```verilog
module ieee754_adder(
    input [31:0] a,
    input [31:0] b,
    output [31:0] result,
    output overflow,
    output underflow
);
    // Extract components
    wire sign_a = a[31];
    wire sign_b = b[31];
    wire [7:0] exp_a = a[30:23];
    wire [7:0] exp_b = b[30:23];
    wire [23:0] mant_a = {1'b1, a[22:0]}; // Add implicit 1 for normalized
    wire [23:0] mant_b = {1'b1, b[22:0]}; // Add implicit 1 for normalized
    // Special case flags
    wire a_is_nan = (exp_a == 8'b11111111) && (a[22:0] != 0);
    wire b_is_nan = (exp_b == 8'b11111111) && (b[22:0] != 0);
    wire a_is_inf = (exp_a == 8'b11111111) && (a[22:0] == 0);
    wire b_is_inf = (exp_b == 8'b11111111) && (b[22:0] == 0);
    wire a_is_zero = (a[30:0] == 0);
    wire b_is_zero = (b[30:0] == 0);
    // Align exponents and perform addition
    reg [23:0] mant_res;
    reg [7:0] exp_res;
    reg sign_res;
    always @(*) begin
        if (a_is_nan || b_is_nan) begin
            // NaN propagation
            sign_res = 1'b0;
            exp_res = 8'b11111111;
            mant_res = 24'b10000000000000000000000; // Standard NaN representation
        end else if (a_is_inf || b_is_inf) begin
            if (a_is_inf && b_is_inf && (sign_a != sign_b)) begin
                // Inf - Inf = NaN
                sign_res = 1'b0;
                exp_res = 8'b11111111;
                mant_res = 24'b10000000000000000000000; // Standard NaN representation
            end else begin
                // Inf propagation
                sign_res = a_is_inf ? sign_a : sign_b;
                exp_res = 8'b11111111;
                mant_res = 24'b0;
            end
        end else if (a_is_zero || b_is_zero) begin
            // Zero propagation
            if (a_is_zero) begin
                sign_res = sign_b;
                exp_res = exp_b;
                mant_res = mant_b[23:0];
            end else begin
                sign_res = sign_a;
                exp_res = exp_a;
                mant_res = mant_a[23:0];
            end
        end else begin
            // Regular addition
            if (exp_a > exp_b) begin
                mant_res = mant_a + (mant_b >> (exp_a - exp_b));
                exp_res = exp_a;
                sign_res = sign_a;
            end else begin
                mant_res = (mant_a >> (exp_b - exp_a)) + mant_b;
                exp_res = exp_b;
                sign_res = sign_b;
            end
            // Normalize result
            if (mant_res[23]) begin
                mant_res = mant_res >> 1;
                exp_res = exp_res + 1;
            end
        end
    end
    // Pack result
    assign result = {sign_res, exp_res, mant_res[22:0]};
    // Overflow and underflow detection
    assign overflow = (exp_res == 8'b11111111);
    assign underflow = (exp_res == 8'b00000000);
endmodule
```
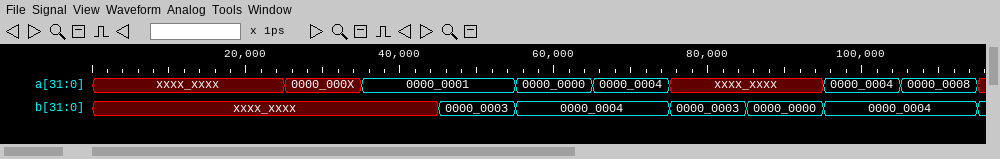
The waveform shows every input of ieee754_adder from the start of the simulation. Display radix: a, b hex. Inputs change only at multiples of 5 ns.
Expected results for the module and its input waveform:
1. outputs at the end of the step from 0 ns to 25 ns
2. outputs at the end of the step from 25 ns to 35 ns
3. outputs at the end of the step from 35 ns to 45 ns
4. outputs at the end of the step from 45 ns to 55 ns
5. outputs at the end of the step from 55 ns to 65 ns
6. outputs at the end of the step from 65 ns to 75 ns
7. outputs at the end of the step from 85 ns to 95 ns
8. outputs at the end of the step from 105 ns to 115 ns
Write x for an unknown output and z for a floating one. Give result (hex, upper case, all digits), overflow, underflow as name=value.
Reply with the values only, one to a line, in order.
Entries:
result=x, overflow=x, underflow=x
result=x, overflow=x, underflow=x
result=x, overflow=x, underflow=x
result=00000004, overflow=0, underflow=1
result=00000004, overflow=0, underflow=1
result=00000008, overflow=0, underflow=1
result=x, overflow=x, underflow=x
result=0000000C, overflow=0, underflow=1
